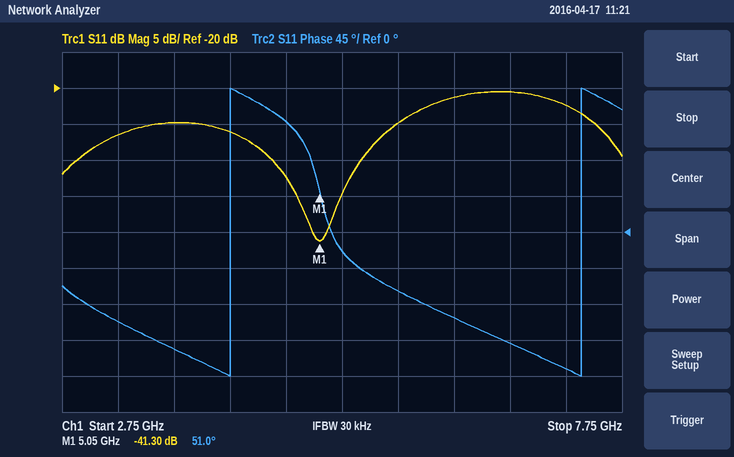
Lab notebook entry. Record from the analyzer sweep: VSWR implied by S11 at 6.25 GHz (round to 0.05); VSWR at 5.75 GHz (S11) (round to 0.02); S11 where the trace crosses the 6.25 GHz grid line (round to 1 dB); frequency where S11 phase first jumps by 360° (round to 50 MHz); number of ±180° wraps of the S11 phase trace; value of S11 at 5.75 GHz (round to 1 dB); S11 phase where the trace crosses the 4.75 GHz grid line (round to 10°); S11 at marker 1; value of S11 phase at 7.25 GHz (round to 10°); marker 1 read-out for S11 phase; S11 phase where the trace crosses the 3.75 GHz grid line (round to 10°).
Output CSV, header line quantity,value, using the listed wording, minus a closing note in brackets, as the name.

quantity,value
VSWR implied by S11 at 6.25 GHz,1.20
VSWR at 5.75 GHz (S11),1.12
S11 where the trace crosses the 6.25 GHz grid line,-21 dB
frequency where S11 phase first jumps by 360°,4.25 GHz
number of ±180° wraps of the S11 phase trace,2
value of S11 at 5.75 GHz,-25 dB
S11 phase where the trace crosses the 4.75 GHz grid line,140°
S11 at marker 1,-41.30 dB
value of S11 phase at 7.25 GHz,-170°
marker 1 read-out for S11 phase,51.0°
S11 phase where the trace crosses the 3.75 GHz grid line,-150°
